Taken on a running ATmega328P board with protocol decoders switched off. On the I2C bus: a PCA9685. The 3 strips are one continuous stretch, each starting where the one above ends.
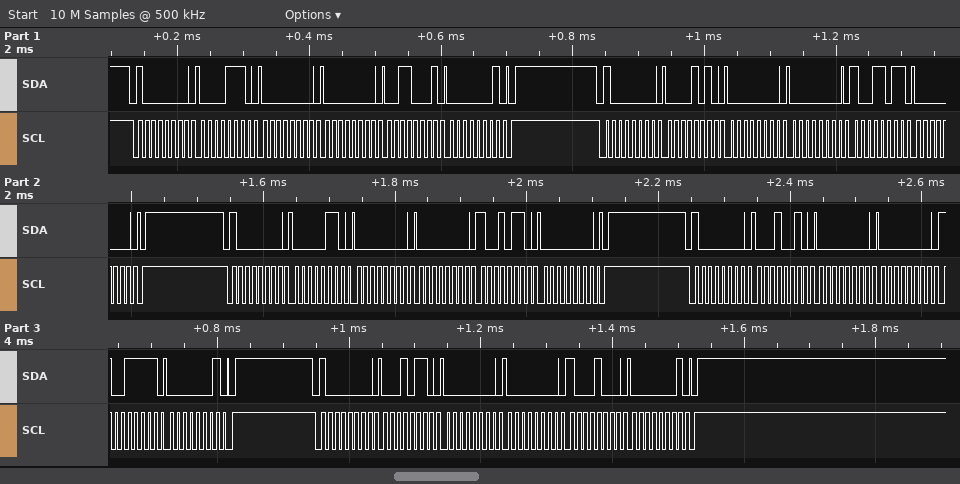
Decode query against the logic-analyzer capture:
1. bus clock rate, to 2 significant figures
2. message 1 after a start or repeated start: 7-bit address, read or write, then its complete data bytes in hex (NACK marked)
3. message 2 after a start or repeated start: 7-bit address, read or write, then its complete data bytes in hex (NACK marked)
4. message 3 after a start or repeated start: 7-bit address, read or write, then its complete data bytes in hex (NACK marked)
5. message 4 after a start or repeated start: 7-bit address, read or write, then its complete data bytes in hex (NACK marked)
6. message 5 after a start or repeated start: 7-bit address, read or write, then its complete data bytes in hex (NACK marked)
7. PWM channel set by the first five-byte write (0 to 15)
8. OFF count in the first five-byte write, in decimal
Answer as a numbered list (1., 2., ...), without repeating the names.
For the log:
1. 100 kHz
2. 0x40 write: 0E 00 00 31 01
3. 0x40 write: 0A 00 00 9B 00
4. 0x40 write: 06 00 00 96 00
5. 0x40 write: 12 00 00 9F 01
6. 0x40 write: 16 00 00 88 01
7. 2
8. 305
